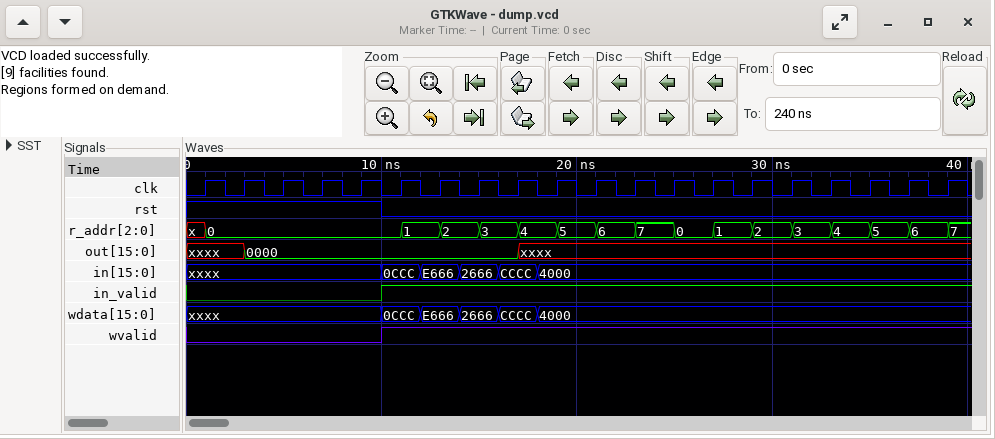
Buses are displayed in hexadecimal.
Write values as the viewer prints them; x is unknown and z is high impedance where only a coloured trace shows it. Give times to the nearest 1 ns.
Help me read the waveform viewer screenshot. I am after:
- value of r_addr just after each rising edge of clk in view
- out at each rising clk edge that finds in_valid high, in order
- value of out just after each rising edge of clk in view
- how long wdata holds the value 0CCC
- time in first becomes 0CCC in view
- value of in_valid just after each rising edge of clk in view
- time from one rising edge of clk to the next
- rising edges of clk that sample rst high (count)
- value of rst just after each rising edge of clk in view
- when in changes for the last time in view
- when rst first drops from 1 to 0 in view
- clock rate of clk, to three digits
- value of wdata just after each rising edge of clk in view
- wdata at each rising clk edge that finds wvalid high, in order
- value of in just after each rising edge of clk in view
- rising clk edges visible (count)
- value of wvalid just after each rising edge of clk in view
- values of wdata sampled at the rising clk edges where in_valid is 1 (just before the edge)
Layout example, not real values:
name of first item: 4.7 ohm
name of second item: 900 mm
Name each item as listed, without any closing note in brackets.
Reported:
value of r_addr just after each rising edge of clk in view: 0, 0, 0, 0, 0, 1, 2, 3, 4, 5, 6, 7, 0, 1, 2, 3, 4, 5, 6, 7
out at each rising clk edge that finds in_valid high, in order: 0000, 0000, 0000, 0000, xxxx, xxxx, xxxx, xxxx, xxxx, xxxx, xxxx, xxxx, xxxx, xxxx, xxxx
value of out just after each rising edge of clk in view: xxxx, 0000, 0000, 0000, 0000, 0000, 0000, 0000, xxxx, xxxx, xxxx, xxxx, xxxx, xxxx, xxxx, xxxx, xxxx, xxxx, xxxx, xxxx
how long wdata holds the value 0CCC: 2 ns
time in first becomes 0CCC in view: 10 ns
value of in_valid just after each rising edge of clk in view: 0 0 0 0 0 1 1 1 1 1 1 1 1 1 1 1 1 1 1 1
time from one rising edge of clk to the next: 2 ns
rising edges of clk that sample rst high: 5
value of rst just after each rising edge of clk in view: 1 1 1 1 1 0 0 0 0 0 0 0 0 0 0 0 0 0 0 0
when in changes for the last time in view: 18 ns
when rst first drops from 1 to 0 in view: 10 ns
clock rate of clk, to three digits: 500 MHz
value of wdata just after each rising edge of clk in view: xxxx, xxxx, xxxx, xxxx, xxxx, 0CCC, E666, 2666, CCCC, 4000, 4000, 4000, 4000, 4000, 4000, 4000, 4000, 4000, 4000, 4000
wdata at each rising clk edge that finds wvalid high, in order: 0CCC, E666, 2666, CCCC, 4000, 4000, 4000, 4000, 4000, 4000, 4000, 4000, 4000, 4000, 4000
value of in just after each rising edge of clk in view: xxxx, xxxx, xxxx, xxxx, xxxx, 0CCC, E666, 2666, CCCC, 4000, 4000, 4000, 4000, 4000, 4000, 4000, 4000, 4000, 4000, 4000
rising clk edges visible: 20
value of wvalid just after each rising edge of clk in view: 0 0 0 0 0 1 1 1 1 1 1 1 1 1 1 1 1 1 1 1
values of wdata sampled at the rising clk edges where in_valid is 1: 0CCC, E666, 2666, CCCC, 4000, 4000, 4000, 4000, 4000, 4000, 4000, 4000, 4000, 4000, 4000
